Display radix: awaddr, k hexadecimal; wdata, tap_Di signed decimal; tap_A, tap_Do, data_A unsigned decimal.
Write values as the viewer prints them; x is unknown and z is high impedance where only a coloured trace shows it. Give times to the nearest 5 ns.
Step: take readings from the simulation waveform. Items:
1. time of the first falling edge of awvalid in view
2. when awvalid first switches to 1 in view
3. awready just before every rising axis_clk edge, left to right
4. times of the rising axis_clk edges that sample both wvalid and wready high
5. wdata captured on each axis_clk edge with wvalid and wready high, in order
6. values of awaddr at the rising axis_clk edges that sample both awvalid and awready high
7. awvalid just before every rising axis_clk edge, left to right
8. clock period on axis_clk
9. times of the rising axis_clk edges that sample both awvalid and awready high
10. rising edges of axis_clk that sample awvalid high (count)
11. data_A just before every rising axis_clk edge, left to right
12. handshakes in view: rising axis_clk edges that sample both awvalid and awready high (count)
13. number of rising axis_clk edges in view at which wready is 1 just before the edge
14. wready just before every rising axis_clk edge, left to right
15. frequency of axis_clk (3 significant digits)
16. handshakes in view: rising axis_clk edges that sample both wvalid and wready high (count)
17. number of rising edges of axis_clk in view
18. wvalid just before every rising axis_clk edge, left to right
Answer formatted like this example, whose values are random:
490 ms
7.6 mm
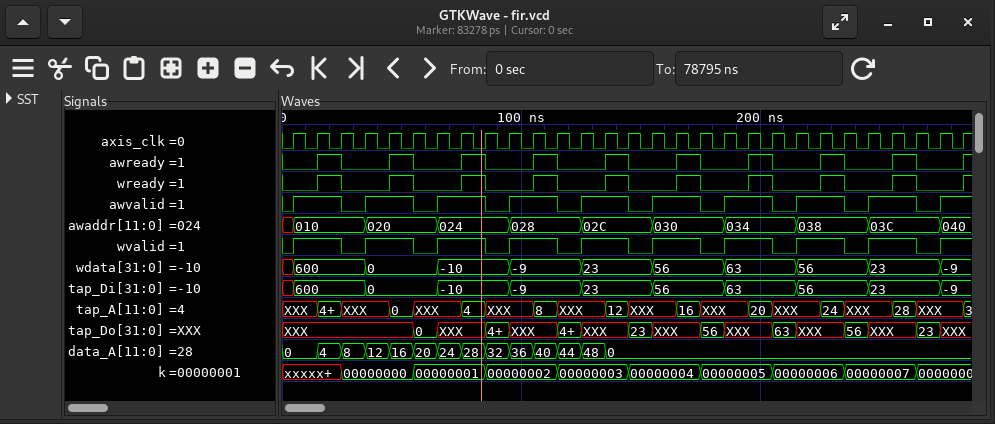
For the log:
25 ns
5 ns
0 0 1 0 0 1 0 0 1 0 0 1 0 0 1 0 0 1 0 0 1 0 0 1 0 0 1 0 0
25 ns, 55 ns, 85 ns, 115 ns, 145 ns, 175 ns, 205 ns, 235 ns, 265 ns
600, 0, -10, -9, 23, 56, 63, 56, 23
010, 020, 024, 028, 02C, 030, 034, 038, 03C
0 1 1 0 1 1 0 1 1 0 1 1 0 1 1 0 1 1 0 1 1 0 1 1 0 1 1 0 1
10 ns
25 ns, 55 ns, 85 ns, 115 ns, 145 ns, 175 ns, 205 ns, 235 ns, 265 ns
19
0, 0, 4, 8, 12, 16, 20, 24, 28, 32, 36, 40, 44, 48, 0, 0, 0, 0, 0, 0, 0, 0, 0, 0, 0, 0, 0, 0, 0
9
9
0 0 1 0 0 1 0 0 1 0 0 1 0 0 1 0 0 1 0 0 1 0 0 1 0 0 1 0 0
100 MHz
9
29
0 1 1 0 1 1 0 1 1 0 1 1 0 1 1 0 1 1 0 1 1 0 1 1 0 1 1 0 1
